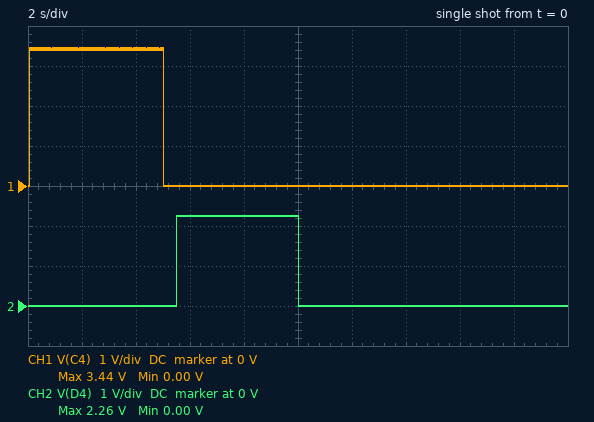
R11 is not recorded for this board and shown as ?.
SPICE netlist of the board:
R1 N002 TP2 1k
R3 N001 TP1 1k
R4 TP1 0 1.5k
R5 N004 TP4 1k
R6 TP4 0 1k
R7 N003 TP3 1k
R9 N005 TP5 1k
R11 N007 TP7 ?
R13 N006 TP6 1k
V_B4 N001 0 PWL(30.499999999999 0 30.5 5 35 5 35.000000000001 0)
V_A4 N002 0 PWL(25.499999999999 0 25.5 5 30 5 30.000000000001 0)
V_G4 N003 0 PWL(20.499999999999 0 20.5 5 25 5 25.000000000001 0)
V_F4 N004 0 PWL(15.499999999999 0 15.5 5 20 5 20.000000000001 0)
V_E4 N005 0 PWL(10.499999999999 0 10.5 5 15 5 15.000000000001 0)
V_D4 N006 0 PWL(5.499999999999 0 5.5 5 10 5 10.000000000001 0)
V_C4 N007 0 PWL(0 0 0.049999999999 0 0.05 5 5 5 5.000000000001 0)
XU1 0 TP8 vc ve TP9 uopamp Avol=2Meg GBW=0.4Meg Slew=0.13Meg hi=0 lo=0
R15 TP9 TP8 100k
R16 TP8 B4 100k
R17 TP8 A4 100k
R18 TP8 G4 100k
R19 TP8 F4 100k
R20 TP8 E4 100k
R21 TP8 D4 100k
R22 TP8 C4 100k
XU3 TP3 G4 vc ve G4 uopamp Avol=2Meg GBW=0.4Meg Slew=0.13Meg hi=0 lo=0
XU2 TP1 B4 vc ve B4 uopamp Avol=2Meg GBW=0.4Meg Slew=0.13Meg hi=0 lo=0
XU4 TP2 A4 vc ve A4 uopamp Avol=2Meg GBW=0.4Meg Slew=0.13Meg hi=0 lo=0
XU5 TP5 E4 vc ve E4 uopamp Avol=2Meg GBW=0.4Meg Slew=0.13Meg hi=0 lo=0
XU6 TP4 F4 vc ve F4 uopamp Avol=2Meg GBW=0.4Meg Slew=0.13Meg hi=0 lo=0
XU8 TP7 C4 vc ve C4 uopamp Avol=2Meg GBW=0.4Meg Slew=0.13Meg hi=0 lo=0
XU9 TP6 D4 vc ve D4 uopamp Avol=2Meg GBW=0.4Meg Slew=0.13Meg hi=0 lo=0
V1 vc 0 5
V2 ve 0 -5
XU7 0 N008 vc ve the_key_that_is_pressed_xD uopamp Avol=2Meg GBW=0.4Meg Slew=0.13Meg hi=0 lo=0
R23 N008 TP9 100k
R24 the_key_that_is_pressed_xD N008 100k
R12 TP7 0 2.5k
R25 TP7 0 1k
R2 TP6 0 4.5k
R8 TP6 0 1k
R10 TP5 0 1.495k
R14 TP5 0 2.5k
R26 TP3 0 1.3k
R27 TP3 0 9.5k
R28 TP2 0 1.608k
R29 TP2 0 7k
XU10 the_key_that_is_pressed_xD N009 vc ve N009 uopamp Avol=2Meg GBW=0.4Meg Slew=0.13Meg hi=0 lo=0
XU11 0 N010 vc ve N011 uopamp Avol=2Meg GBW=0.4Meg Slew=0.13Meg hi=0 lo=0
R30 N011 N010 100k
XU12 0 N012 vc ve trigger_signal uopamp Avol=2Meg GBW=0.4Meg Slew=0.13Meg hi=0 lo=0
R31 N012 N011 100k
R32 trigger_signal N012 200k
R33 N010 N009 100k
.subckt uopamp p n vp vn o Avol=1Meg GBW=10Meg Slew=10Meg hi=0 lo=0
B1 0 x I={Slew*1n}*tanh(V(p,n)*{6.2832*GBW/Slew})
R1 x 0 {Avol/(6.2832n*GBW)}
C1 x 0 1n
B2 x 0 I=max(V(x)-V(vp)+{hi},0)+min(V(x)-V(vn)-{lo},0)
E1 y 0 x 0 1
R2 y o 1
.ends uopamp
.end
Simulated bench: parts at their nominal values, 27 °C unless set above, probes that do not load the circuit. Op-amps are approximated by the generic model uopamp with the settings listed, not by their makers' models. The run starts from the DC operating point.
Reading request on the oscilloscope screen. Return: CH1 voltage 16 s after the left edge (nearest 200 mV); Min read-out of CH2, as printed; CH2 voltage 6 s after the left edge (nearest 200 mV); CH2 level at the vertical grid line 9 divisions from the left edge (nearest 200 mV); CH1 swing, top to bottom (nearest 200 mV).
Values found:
0 V
0.00 V
2.2 V
0 V
3.4 V
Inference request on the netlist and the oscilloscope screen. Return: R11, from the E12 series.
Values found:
330 Ω
